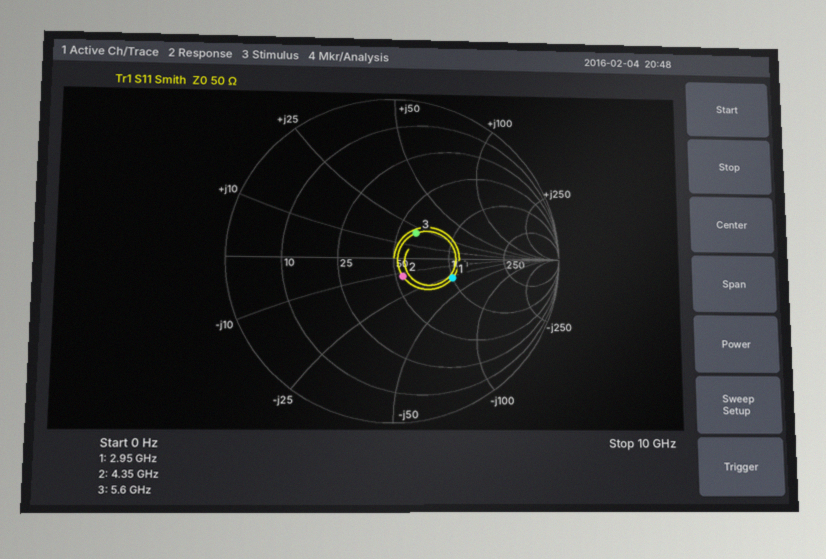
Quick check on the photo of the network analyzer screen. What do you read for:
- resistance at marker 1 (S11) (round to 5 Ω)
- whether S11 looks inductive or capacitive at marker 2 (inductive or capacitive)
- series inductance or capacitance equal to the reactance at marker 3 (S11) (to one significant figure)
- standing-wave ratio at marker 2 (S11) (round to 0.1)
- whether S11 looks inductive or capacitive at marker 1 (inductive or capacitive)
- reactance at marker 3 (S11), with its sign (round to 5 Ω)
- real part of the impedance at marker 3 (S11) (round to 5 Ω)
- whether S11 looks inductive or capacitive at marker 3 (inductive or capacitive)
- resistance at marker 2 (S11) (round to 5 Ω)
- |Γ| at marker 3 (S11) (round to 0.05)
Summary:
100 Ω
capacitive
600 pH
1.3
capacitive
+20 Ω
60 Ω
inductive
55 Ω
0.20
